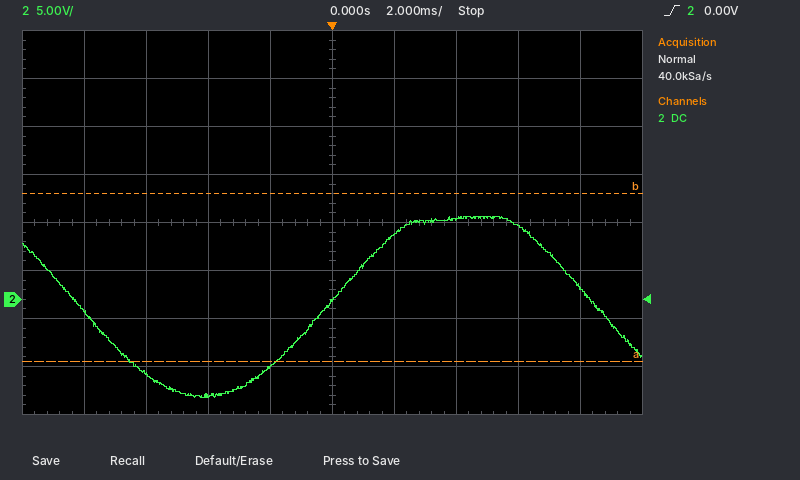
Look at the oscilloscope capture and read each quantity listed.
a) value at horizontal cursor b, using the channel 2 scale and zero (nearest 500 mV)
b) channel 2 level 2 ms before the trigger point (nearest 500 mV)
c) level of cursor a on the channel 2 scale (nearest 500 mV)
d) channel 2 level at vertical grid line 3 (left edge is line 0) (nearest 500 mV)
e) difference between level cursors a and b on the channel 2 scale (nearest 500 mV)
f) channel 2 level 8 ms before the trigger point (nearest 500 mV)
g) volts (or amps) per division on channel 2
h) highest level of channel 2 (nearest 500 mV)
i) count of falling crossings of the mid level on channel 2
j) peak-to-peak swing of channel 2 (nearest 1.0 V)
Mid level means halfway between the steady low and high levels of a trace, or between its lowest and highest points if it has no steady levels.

11.0 V
-7.0 V
-6.5 V
-10.0 V
17.5 V
-1.5 V
5 V
8.5 V
2
19.0 V
